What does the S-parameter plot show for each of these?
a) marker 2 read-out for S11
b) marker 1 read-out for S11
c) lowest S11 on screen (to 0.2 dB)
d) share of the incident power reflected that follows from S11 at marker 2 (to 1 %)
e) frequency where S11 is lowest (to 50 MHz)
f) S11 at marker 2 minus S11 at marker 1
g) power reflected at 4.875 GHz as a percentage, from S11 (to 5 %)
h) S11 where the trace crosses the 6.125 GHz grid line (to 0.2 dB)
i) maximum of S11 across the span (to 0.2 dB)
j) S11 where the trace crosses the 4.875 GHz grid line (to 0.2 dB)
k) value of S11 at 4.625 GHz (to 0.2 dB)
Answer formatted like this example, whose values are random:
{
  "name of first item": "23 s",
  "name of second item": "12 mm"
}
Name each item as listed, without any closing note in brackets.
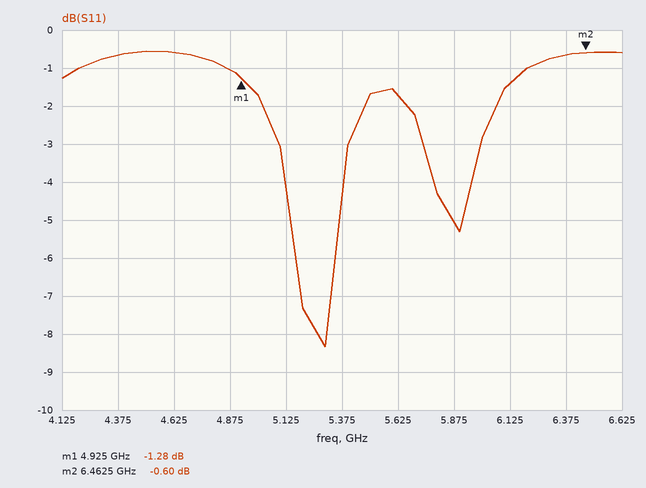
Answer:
{
  "marker 2 read-out for S11": "-0.60 dB",
  "marker 1 read-out for S11": "-1.28 dB",
  "lowest S11 on screen": "-8.4 dB",
  "share of the incident power reflected that follows from S11 at marker 2": "87 %",
  "frequency where S11 is lowest": "5.30 GHz",
  "S11 at marker 2 minus S11 at marker 1": "0.68 dB",
  "power reflected at 4.875 GHz as a percentage, from S11": "80 %",
  "S11 where the trace crosses the 6.125 GHz grid line": "-1.4 dB",
  "maximum of S11 across the span": "-0.6 dB",
  "S11 where the trace crosses the 4.875 GHz grid line": "-1.0 dB",
  "value of S11 at 4.625 GHz": "-0.6 dB"
}
